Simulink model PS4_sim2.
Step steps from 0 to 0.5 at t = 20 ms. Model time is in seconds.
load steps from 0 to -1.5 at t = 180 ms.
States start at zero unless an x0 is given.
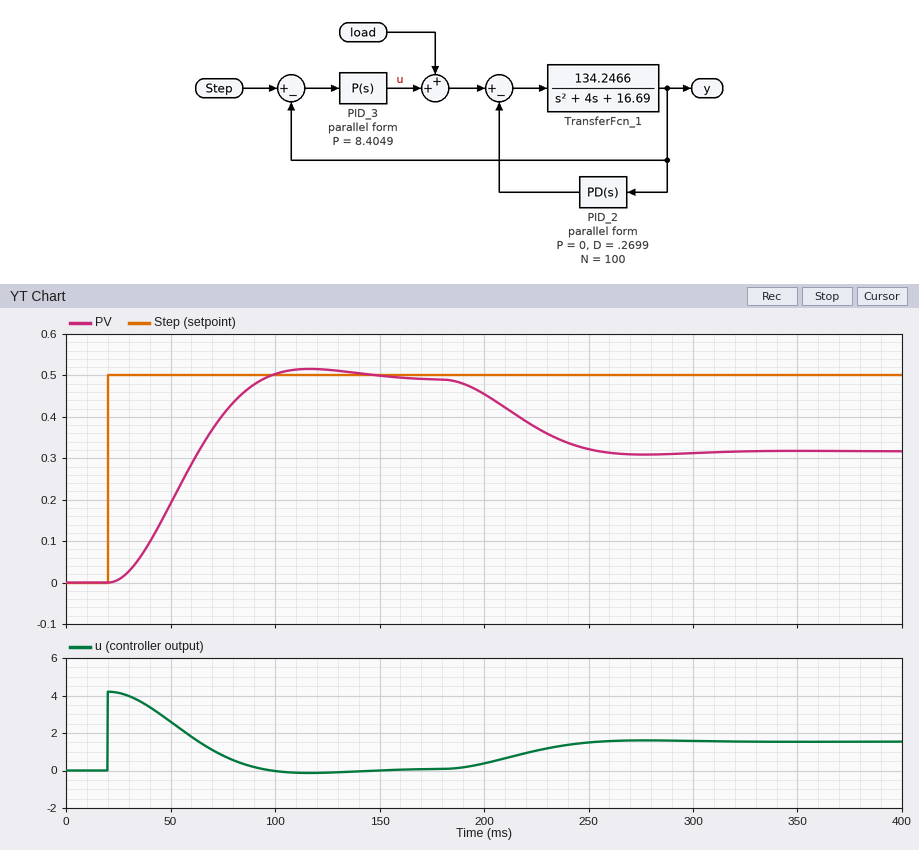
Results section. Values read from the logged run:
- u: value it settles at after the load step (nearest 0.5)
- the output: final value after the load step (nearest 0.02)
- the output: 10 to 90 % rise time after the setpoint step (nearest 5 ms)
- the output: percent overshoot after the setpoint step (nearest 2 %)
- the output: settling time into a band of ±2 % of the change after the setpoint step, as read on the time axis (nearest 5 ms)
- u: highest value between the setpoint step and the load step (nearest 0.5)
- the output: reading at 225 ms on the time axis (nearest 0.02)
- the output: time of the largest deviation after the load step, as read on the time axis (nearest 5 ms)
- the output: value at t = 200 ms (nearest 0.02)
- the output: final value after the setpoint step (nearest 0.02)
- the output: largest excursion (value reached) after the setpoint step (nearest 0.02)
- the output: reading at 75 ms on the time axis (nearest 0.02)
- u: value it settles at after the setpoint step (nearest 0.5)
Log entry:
1.5
0.32
50 ms
4 %
145 ms
4.0
0.38
275 ms
0.46
0.50
0.52
0.40
0.0
